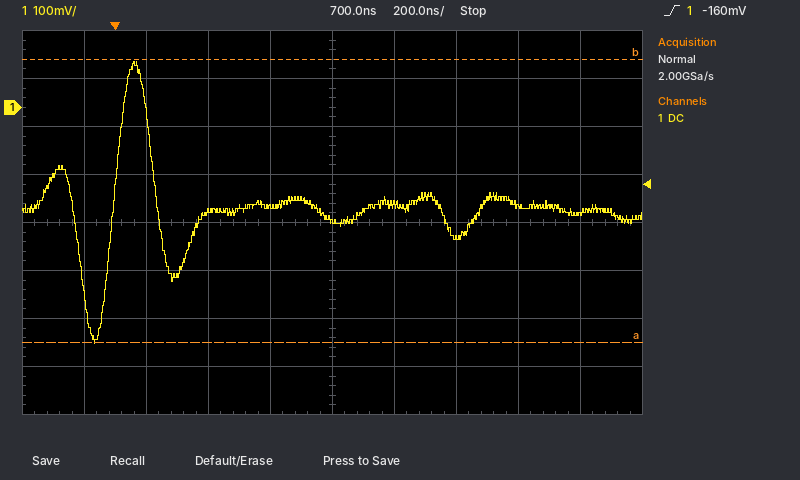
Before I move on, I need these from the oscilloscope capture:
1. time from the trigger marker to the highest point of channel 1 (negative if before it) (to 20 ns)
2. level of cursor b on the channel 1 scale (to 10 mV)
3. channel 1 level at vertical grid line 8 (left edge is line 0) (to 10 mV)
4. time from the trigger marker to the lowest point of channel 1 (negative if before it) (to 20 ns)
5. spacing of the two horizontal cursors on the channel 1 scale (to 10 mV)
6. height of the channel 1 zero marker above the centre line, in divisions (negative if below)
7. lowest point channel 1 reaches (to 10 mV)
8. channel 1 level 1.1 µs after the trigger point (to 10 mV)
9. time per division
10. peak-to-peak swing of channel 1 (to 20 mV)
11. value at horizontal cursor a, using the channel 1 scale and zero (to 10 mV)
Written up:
+60 ns
100 mV
-200 mV
-60 ns
590 mV
+2.4 div
-490 mV
-270 mV
200 ns
580 mV
-490 mV
